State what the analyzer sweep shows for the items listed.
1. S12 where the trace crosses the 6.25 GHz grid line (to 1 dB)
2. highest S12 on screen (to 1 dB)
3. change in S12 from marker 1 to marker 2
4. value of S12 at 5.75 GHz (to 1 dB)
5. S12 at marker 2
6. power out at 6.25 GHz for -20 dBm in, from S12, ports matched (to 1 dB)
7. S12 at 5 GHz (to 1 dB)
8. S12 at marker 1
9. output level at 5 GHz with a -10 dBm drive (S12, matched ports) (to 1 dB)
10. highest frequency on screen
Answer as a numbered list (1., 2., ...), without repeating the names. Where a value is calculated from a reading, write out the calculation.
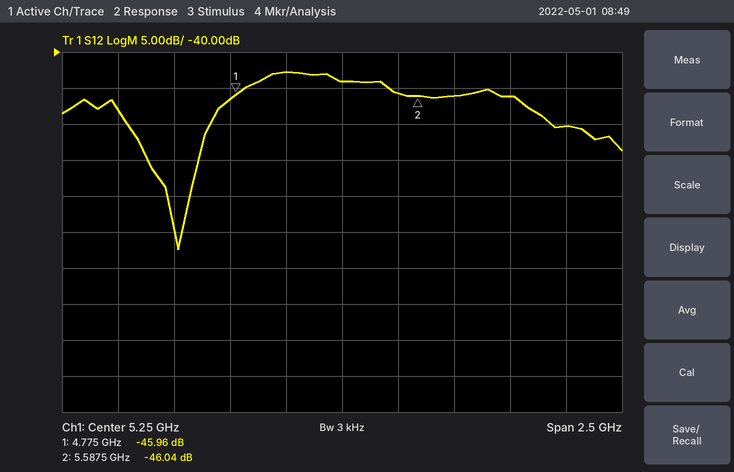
1. -50 dB
2. -43 dB
3. -46.04 − (-45.96) = -0.08 dB
4. -46 dB
5. -46.04 dB
6. -20 dBm + (-50 dB) = -70 dBm
7. -43 dB
8. -45.96 dB
9. -10 dBm + (-43 dB) = -53 dBm
10. 6.5 GHz
